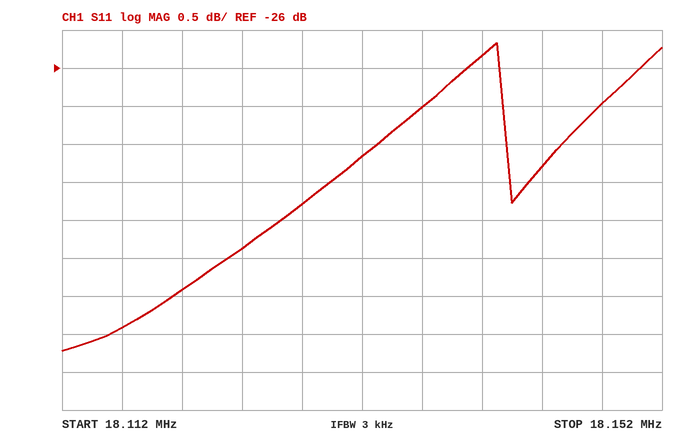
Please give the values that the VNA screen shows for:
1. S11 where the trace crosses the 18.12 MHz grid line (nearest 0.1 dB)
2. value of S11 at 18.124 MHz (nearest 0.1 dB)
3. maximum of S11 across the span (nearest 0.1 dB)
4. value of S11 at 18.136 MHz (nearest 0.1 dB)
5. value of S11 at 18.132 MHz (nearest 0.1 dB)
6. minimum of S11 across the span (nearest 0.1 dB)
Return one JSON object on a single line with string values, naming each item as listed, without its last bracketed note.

{"S11 where the trace crosses the 18.12 MHz grid line": "-28.9 dB", "value of S11 at 18.124 MHz": "-28.4 dB", "maximum of S11 across the span": "-25.7 dB", "value of S11 at 18.136 MHz": "-26.5 dB", "value of S11 at 18.132 MHz": "-27.2 dB", "minimum of S11 across the span": "-29.7 dB"}
